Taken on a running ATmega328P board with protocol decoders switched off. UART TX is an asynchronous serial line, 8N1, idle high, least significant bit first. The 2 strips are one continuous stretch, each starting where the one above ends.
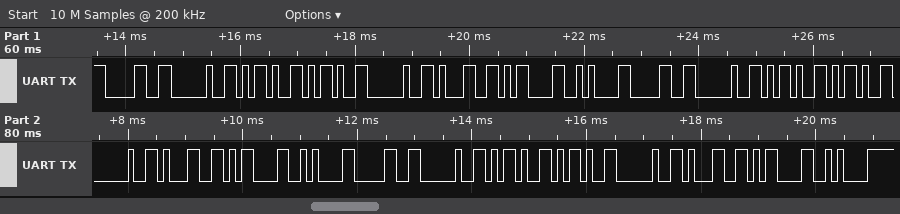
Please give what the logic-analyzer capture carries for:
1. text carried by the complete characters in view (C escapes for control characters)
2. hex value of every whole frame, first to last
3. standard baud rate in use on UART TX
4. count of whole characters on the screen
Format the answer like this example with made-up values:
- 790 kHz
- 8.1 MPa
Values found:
- "0 -- 1\r\n0 -- 1\r\n0 -- 1\r\n"
- 30 20 2D 2D 20 31 0D 0A 30 20 2D 2D 20 31 0D 0A 30 20 2D 2D 20 31 0D 0A
- 9600 baud
- 24
